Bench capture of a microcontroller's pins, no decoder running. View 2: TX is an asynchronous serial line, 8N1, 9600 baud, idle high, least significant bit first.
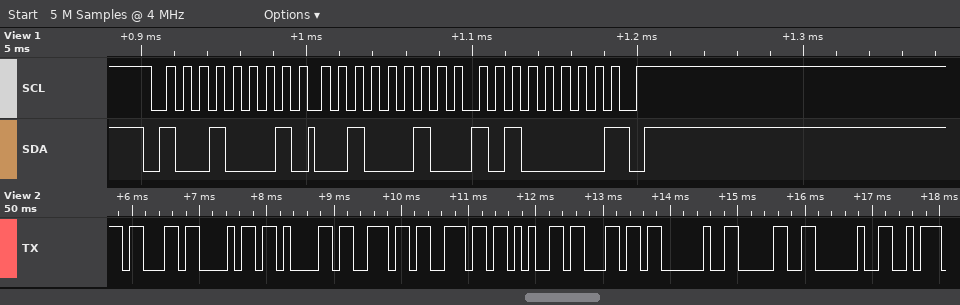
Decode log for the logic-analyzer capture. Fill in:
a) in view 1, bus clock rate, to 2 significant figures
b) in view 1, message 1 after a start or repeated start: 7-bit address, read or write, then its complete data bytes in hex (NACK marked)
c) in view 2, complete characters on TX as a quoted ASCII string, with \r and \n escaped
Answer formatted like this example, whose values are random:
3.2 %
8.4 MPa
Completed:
100 kHz
0x48 read: 22 A0 NACK
"channel 0 "
